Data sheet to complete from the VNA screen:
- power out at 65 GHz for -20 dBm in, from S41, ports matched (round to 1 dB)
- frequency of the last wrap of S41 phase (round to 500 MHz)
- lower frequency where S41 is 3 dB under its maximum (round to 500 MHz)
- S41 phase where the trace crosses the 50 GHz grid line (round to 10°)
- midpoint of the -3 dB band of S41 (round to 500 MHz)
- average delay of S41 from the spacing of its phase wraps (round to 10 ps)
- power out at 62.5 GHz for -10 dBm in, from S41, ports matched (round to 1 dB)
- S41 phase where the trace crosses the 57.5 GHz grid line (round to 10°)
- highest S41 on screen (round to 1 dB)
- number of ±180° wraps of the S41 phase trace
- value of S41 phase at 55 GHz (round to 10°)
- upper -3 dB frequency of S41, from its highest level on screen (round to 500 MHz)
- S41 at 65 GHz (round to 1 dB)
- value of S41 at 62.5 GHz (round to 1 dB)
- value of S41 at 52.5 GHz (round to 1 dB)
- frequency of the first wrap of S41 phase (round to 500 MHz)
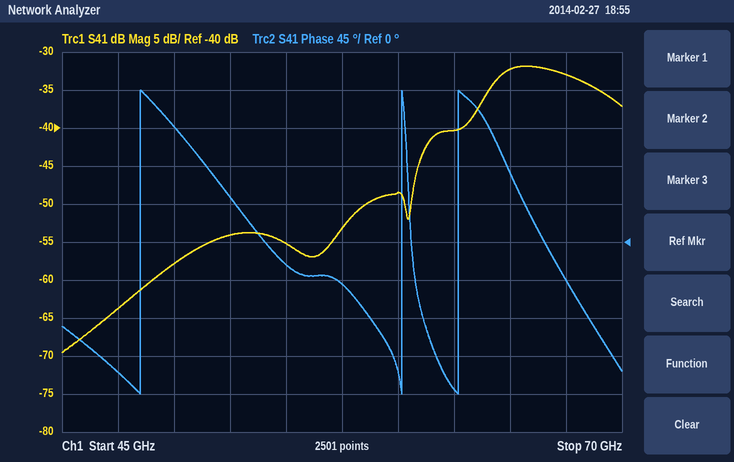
-52 dBm
62.5 GHz
64.0 GHz
140°
66.5 GHz
140 ps
-50 dBm
-50°
-32 dB
3
-30°
69.0 GHz
-32 dB
-40 dB
-54 dB
48.5 GHz
